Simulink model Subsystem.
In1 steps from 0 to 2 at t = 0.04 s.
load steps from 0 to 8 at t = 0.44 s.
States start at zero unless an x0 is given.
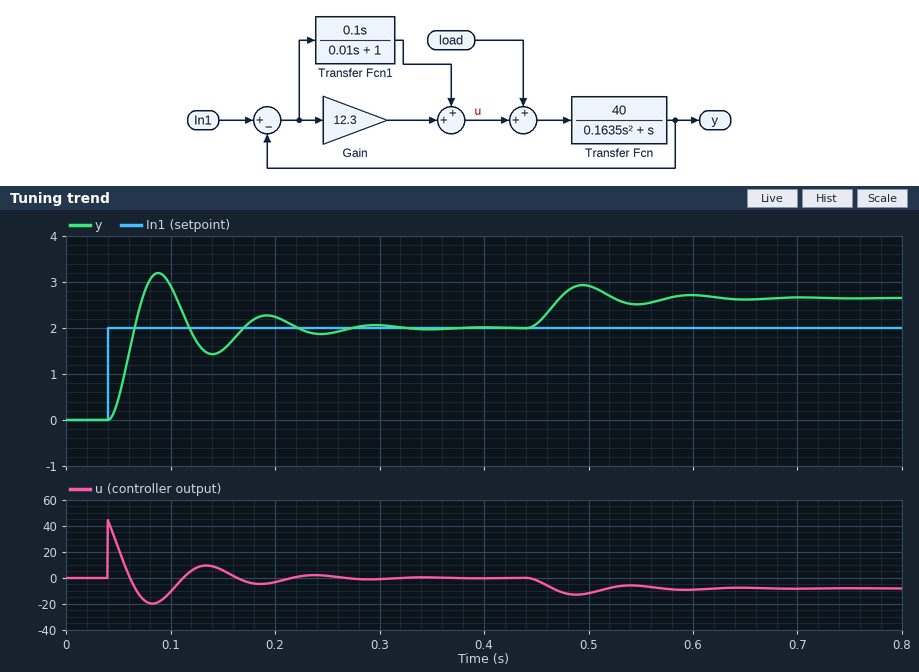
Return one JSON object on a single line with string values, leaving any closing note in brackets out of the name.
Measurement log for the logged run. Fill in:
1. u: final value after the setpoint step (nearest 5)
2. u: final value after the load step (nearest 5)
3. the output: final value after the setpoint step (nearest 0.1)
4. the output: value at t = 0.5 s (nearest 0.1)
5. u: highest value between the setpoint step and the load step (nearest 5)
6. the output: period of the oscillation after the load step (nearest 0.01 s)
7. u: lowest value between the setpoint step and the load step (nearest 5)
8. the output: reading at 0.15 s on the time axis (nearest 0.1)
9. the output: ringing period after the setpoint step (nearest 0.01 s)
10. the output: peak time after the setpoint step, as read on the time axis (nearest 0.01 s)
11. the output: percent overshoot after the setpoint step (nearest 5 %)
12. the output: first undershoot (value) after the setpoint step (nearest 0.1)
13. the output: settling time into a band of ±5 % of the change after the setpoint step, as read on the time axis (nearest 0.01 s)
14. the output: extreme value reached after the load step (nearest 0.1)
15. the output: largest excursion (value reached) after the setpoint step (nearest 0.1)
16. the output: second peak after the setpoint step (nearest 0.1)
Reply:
{"u: final value after the setpoint step": "0", "u: final value after the load step": "-10", "the output: final value after the setpoint step": "2.0", "the output: value at t = 0.5 s": "2.9", "u: highest value between the setpoint step and the load step": "45", "the output: period of the oscillation after the load step": "0.10 s", "u: lowest value between the setpoint step and the load step": "-20", "the output: reading at 0.15 s on the time axis": "1.5", "the output: ringing period after the setpoint step": "0.10 s", "the output: peak time after the setpoint step, as read on the time axis": "0.09 s", "the output: percent overshoot after the setpoint step": "60 %", "the output: first undershoot (value) after the setpoint step": "1.4", "the output: settling time into a band of ±5 % of the change after the setpoint step, as read on the time axis": "0.26 s", "the output: extreme value reached after the load step": "2.9", "the output: largest excursion (value reached) after the setpoint step": "3.2", "the output: second peak after the setpoint step": "2.3"}
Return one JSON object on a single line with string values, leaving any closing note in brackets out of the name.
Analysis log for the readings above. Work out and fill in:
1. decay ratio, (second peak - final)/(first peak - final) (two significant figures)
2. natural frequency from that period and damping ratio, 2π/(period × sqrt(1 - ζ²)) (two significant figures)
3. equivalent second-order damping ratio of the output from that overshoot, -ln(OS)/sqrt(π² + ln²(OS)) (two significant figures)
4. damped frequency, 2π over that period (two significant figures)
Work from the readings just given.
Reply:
{"decay ratio, (second peak - final)/(first peak - final)": "0.25", "natural frequency from that period and damping ratio, 2π/(period × sqrt(1 - ζ²))": "64 rad/s", "equivalent second-order damping ratio of the output from that overshoot, -ln(OS)/sqrt(π² + ln²(OS))": "0.16", "damped frequency, 2π over that period": "63 rad/s"}
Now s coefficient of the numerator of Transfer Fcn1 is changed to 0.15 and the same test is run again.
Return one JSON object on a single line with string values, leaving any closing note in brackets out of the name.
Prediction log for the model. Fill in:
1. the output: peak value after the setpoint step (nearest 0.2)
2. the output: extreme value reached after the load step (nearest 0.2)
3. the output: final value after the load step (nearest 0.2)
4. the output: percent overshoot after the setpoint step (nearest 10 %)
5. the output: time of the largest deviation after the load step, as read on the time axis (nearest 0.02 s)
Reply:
{"the output: peak value after the setpoint step": "3.0", "the output: extreme value reached after the load step": "2.8", "the output: final value after the load step": "2.6", "the output: percent overshoot after the setpoint step": "50 %", "the output: time of the largest deviation after the load step, as read on the time axis": "0.50 s"}
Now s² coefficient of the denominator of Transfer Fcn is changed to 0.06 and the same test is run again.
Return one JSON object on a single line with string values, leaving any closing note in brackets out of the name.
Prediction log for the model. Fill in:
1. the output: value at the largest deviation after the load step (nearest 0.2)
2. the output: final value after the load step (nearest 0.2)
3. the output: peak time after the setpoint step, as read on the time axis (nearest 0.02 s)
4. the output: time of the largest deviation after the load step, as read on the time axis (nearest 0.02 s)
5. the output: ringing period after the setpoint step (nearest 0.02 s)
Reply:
{"the output: value at the largest deviation after the load step": "2.8", "the output: final value after the load step": "2.6", "the output: peak time after the setpoint step, as read on the time axis": "0.06 s", "the output: time of the largest deviation after the load step, as read on the time axis": "0.48 s", "the output: ringing period after the setpoint step": "0.06 s"}
